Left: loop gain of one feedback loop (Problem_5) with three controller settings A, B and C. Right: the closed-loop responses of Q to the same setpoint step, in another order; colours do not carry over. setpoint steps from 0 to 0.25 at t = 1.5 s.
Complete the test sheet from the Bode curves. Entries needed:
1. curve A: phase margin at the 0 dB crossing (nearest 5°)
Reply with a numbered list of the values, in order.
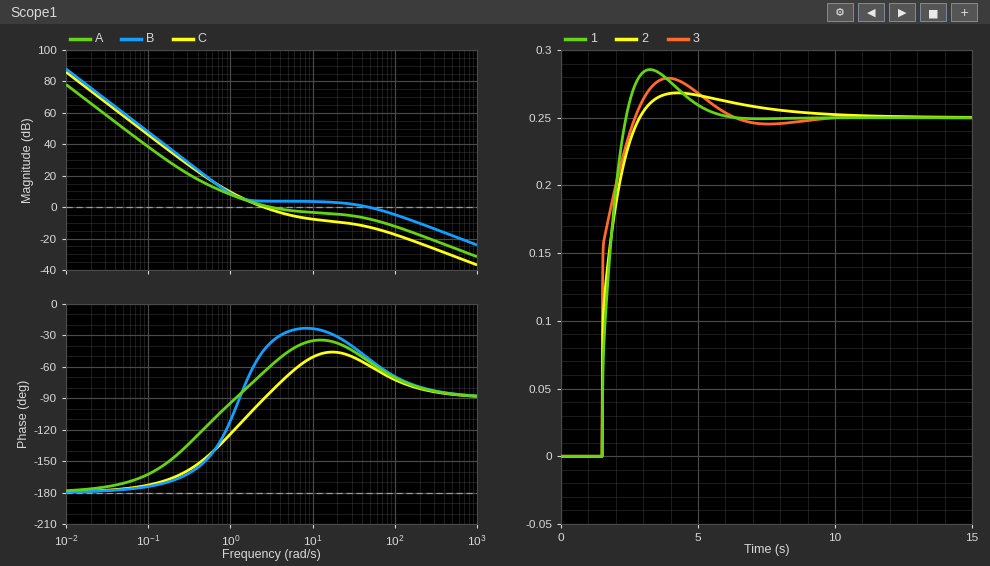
1. 120°
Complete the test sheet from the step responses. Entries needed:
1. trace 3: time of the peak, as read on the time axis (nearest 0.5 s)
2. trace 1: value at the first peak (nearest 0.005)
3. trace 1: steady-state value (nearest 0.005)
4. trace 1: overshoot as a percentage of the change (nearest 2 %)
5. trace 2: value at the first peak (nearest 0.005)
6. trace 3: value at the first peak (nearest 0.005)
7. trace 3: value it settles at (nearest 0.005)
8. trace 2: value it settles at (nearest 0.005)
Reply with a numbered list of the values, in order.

1. 4.0 s
2. 0.285
3. 0.250
4. 14 %
5. 0.270
6. 0.280
7. 0.250
8. 0.250
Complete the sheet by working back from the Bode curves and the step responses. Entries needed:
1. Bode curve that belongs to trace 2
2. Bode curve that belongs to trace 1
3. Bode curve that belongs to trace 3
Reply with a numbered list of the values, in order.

1. A
2. C
3. B
